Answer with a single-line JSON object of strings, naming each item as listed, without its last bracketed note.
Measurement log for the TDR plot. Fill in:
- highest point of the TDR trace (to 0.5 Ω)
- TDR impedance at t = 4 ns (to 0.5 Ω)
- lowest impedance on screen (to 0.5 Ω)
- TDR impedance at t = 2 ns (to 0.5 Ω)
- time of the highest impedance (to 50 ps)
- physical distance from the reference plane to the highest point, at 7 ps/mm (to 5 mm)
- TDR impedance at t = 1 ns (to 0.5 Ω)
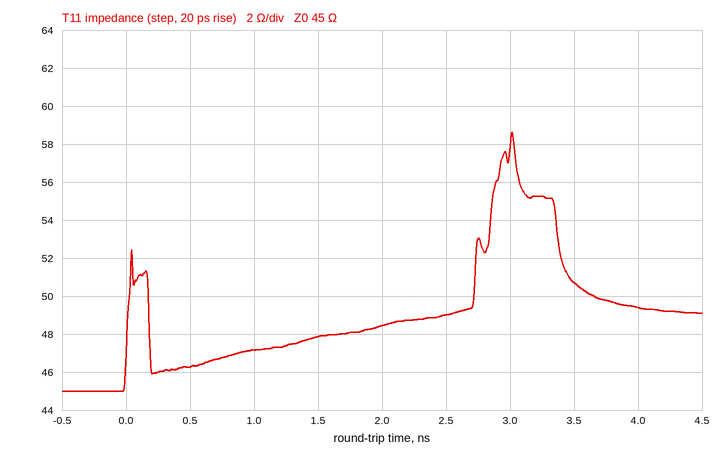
{"highest point of the TDR trace": "58.5 Ω", "TDR impedance at t = 4 ns": "49.5 Ω", "lowest impedance on screen": "45.0 Ω", "TDR impedance at t = 2 ns": "48.5 Ω", "time of the highest impedance": "3.00 ns", "physical distance from the reference plane to the highest point, at 7 ps/mm": "215 mm", "TDR impedance at t = 1 ns": "47.0 Ω"}
